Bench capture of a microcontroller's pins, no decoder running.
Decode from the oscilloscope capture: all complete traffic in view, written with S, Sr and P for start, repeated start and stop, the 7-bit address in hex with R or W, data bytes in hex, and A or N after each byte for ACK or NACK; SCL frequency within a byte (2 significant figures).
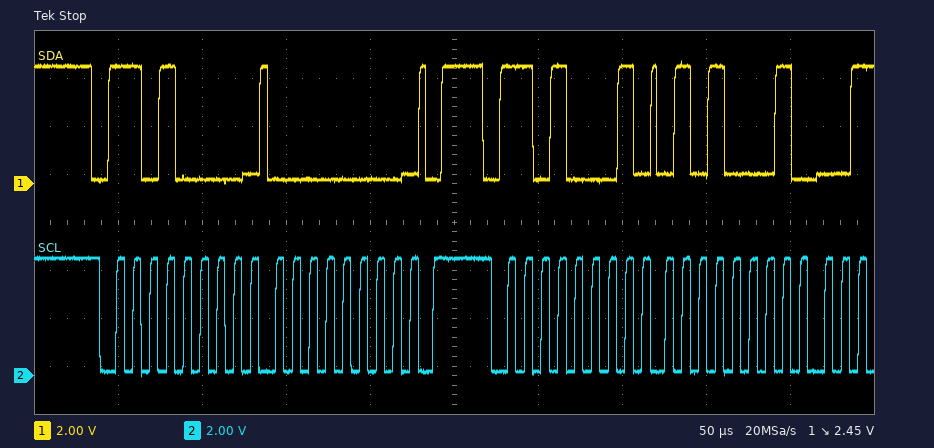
S 68W A 00 A P S 68R A 51 A
100 kHz
